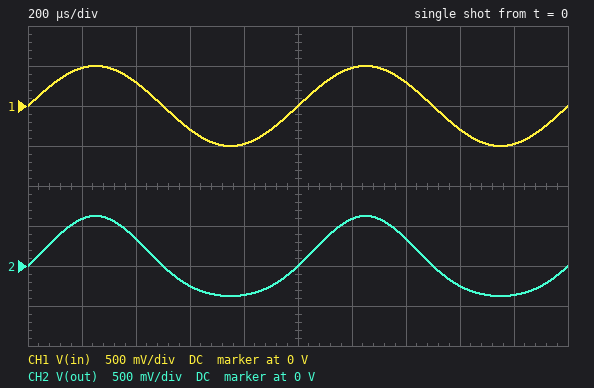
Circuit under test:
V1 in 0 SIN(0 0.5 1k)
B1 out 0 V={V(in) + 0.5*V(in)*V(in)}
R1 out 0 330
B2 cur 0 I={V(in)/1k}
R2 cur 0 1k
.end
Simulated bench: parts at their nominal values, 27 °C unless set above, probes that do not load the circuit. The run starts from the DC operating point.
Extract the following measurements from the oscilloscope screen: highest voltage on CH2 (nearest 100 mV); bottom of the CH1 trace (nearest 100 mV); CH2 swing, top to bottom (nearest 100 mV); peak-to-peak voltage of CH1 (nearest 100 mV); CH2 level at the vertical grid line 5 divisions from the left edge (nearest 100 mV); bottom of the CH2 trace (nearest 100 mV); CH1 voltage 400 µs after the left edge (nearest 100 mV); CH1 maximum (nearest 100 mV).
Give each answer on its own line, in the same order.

600 mV
-500 mV
1.0 V
1.0 V
0 V
-400 mV
300 mV
500 mV
